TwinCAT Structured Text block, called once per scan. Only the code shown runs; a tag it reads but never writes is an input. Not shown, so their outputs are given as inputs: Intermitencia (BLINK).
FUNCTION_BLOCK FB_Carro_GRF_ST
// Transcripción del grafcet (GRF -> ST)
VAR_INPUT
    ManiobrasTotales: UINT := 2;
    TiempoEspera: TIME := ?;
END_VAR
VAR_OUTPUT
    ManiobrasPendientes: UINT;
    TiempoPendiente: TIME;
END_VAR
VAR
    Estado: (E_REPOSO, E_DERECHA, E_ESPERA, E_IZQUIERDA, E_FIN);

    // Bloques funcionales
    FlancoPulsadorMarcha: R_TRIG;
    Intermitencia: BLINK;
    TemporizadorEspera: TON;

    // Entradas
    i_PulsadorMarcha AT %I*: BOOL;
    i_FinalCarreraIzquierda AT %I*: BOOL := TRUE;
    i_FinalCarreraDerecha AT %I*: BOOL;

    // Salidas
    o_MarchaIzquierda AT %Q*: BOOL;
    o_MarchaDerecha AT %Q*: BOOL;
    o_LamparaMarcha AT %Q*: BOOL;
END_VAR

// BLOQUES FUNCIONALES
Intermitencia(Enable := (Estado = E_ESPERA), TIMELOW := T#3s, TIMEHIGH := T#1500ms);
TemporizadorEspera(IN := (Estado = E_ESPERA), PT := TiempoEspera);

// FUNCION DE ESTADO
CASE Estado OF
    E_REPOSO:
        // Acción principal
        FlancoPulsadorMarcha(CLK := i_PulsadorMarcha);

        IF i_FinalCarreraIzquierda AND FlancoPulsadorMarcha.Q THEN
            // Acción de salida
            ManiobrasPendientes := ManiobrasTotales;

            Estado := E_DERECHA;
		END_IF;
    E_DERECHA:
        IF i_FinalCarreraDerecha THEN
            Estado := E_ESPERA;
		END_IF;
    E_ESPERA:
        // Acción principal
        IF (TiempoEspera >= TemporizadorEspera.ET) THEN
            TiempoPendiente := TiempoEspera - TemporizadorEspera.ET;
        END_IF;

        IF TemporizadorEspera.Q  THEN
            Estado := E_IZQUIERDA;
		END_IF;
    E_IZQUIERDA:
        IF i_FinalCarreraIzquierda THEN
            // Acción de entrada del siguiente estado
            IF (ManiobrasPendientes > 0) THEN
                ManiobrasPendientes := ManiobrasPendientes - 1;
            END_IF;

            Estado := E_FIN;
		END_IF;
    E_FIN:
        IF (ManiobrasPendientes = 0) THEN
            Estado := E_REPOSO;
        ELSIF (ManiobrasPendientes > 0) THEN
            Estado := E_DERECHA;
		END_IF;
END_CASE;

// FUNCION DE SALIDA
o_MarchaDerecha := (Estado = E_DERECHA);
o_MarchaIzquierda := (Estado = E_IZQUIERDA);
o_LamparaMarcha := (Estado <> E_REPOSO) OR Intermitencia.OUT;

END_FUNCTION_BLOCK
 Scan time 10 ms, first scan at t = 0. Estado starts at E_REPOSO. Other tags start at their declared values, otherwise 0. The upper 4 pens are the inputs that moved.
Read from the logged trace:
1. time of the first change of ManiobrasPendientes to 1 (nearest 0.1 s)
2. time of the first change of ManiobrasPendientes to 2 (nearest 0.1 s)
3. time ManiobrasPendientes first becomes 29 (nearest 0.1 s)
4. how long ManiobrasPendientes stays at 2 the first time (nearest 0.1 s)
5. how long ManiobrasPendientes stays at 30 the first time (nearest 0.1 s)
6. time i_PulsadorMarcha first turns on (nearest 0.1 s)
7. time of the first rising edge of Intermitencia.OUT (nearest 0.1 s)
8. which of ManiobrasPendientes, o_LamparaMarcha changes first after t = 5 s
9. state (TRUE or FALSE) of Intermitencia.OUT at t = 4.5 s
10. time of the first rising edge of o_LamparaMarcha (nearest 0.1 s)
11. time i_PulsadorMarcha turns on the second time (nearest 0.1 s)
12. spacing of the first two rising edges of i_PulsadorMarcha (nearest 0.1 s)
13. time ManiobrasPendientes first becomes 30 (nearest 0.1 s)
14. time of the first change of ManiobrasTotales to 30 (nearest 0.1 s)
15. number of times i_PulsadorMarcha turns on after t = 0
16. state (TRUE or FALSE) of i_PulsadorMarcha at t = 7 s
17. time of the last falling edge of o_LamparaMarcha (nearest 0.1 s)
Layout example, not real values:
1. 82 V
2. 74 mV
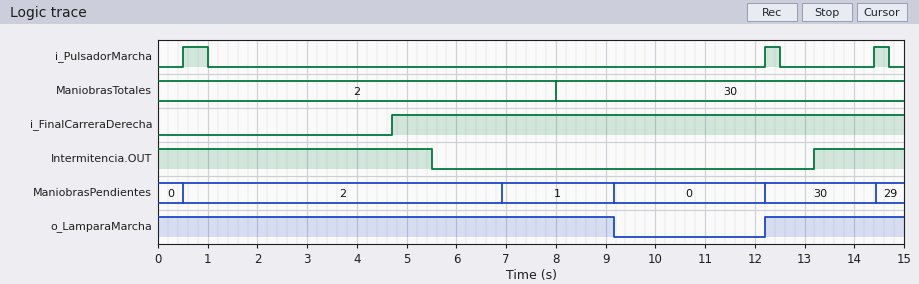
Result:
1. 6.9 s
2. 0.5 s
3. 14.4 s
4. 6.4 s
5. 2.2 s
6. 0.5 s
7. 13.2 s
8. ManiobrasPendientes
9. TRUE
10. 12.2 s
11. 12.2 s
12. 11.7 s
13. 12.2 s
14. 8.0 s
15. 3
16. FALSE
17. 9.2 s
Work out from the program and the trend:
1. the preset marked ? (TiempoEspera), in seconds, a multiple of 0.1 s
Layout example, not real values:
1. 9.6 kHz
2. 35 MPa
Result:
1. 2.2 s
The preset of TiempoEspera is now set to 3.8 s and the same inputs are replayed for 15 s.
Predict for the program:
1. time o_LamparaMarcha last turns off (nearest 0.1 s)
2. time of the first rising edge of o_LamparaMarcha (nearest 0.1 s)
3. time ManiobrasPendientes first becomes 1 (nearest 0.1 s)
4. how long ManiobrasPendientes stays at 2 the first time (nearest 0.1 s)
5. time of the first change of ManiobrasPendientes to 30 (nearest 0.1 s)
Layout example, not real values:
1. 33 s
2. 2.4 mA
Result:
1. 12.4 s
2. 13.2 s
3. 8.5 s
4. 8.0 s
5. 14.4 s
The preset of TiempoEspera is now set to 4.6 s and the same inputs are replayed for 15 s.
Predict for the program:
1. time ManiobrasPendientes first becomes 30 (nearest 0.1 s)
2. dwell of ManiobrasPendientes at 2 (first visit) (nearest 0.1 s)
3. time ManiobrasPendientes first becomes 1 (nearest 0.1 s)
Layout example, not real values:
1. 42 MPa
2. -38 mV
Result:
1. 14.4 s
2. 8.8 s
3. 9.3 s
